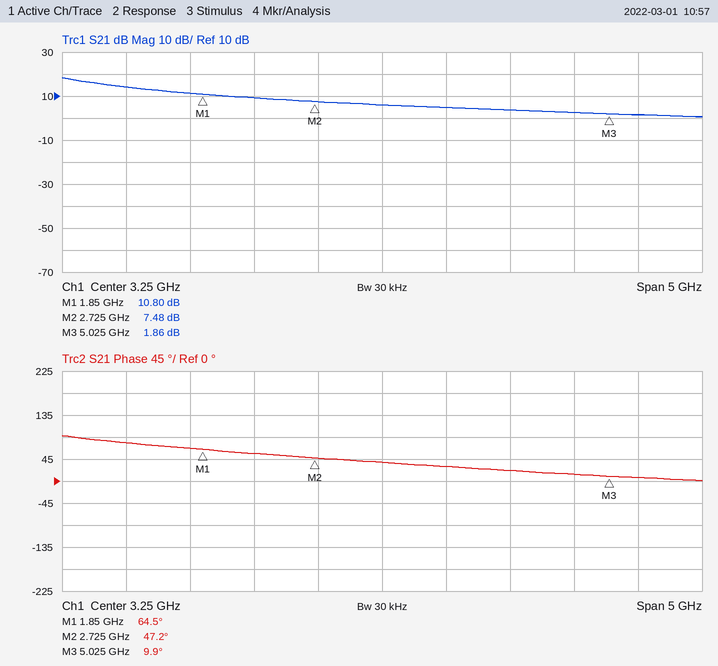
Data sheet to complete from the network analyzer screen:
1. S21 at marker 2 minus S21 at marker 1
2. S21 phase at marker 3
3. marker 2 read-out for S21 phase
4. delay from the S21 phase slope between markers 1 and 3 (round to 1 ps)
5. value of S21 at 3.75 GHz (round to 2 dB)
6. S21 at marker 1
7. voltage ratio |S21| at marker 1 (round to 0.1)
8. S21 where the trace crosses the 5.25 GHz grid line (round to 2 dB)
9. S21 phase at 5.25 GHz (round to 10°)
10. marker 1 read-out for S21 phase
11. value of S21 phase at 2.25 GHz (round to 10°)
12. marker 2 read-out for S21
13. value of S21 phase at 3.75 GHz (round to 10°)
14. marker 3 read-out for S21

-3.32 dB
9.9°
47.2°
48 ps
4 dB
10.80 dB
3.5
2 dB
10°
64.5°
60°
7.48 dB
30°
1.86 dB
